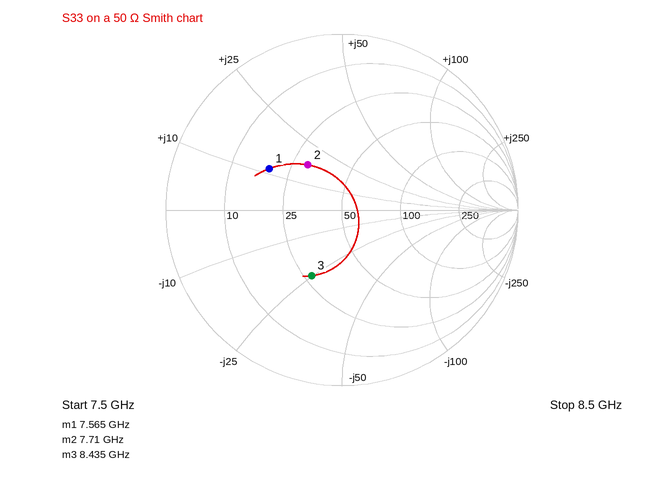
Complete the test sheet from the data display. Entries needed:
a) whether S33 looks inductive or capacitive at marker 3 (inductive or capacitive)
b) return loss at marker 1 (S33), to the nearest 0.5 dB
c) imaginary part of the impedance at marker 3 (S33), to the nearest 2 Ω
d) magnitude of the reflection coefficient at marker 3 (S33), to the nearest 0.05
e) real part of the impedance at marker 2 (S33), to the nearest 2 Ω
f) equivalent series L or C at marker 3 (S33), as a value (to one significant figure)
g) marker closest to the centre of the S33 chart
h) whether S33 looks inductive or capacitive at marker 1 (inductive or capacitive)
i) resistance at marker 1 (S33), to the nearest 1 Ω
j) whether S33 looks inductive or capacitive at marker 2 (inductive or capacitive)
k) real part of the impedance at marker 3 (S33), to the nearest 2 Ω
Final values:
capacitive
6.5 dB
-24 Ω
0.40
30 Ω
800 fF
marker 2
inductive
19 Ω
inductive
28 Ω
